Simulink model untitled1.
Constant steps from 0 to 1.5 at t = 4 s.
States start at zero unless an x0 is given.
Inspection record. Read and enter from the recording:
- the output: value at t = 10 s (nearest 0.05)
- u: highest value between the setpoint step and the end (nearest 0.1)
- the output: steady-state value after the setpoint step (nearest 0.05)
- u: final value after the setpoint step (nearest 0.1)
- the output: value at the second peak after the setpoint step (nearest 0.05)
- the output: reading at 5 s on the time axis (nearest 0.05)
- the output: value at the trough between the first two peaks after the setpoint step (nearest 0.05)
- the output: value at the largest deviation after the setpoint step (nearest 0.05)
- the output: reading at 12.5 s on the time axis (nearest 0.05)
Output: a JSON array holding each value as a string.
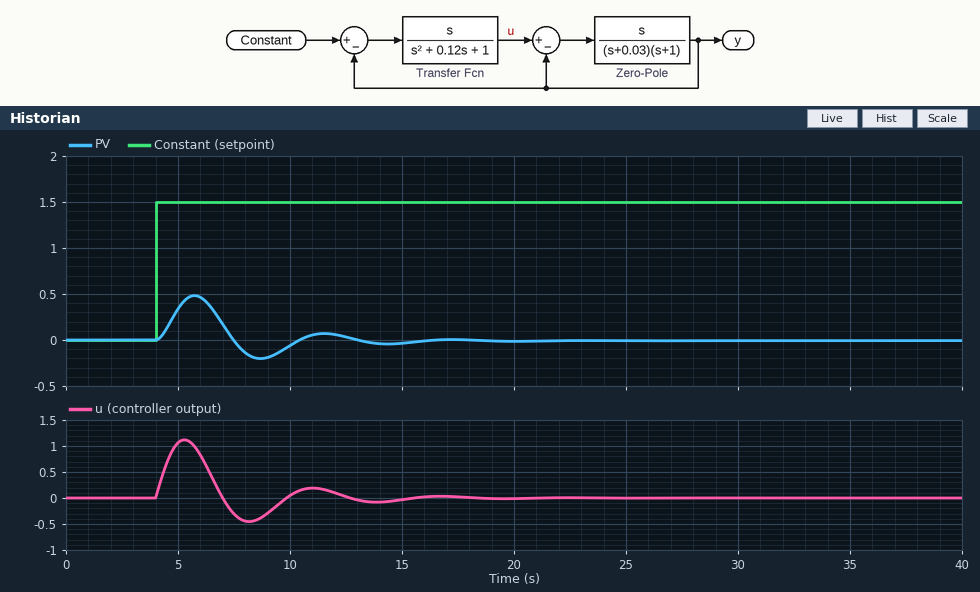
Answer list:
["-0.05", "1.1", "0.00", "0.0", "0.05", "0.35", "-0.20", "0.50", "0.05"]
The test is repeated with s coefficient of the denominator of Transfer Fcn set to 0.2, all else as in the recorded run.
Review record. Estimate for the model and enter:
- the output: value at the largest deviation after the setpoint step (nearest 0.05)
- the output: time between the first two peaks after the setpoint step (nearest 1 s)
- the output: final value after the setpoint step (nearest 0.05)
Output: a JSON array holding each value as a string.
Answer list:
["0.45", "6 s", "0.00"]
